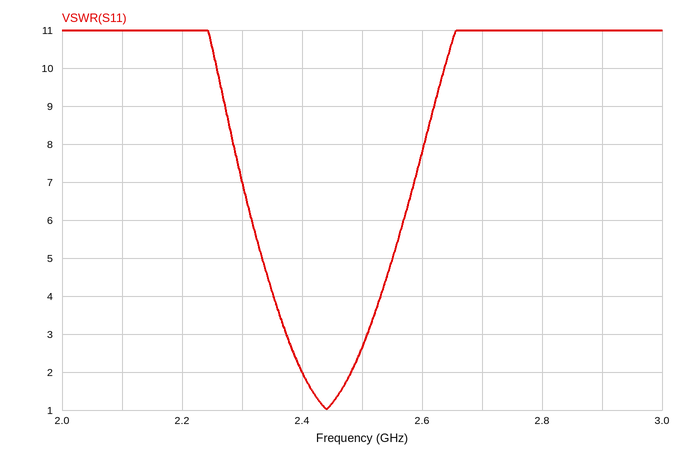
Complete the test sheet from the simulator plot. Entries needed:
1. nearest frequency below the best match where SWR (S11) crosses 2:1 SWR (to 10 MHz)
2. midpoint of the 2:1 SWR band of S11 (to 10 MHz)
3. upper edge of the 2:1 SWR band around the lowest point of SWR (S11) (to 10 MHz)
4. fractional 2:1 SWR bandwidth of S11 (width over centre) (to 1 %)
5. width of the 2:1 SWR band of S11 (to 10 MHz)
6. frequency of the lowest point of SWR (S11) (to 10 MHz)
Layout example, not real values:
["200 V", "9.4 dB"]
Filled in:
["2.40 GHz", "2.44 GHz", "2.48 GHz", "3 %", "80 MHz", "2.44 GHz"]
